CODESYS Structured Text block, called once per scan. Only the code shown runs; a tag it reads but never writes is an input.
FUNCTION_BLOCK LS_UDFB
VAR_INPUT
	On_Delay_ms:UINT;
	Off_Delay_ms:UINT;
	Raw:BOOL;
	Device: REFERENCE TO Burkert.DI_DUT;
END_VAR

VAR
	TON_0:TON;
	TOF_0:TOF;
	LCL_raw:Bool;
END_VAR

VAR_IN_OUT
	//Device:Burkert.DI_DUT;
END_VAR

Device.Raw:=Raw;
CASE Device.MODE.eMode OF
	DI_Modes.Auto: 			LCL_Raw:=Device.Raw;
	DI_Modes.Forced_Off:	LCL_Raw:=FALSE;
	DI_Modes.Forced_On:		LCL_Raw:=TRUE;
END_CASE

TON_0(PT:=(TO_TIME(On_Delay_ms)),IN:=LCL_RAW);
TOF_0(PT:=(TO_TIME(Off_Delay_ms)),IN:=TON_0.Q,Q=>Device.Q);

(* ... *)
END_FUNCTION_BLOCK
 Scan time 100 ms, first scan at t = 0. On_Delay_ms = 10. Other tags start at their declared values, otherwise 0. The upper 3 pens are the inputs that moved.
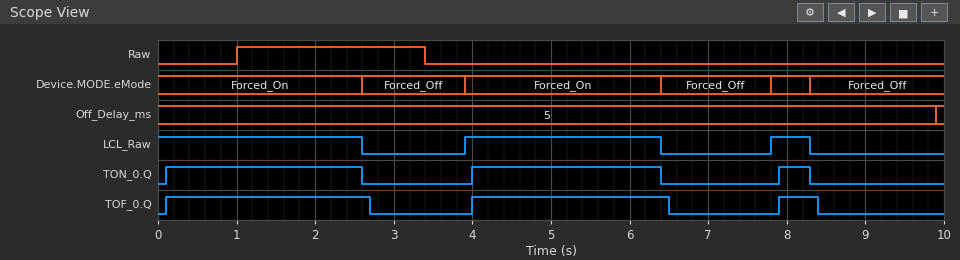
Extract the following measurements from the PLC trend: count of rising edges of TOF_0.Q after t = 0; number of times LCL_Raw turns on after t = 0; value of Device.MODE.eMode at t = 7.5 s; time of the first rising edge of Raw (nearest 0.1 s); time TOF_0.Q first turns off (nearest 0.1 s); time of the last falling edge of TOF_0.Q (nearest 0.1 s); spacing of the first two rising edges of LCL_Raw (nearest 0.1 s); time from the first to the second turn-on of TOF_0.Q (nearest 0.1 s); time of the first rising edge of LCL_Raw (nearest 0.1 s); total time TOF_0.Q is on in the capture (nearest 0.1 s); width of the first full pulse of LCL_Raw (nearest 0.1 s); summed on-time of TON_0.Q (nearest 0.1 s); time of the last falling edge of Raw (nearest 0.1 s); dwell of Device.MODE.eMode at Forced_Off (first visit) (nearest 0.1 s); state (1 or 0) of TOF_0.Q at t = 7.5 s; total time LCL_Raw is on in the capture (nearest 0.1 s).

3
2
Forced_Off
1.0 s
2.7 s
8.4 s
3.9 s
3.9 s
3.9 s
5.6 s
2.5 s
5.3 s
3.4 s
1.3 s
0
5.6 s
